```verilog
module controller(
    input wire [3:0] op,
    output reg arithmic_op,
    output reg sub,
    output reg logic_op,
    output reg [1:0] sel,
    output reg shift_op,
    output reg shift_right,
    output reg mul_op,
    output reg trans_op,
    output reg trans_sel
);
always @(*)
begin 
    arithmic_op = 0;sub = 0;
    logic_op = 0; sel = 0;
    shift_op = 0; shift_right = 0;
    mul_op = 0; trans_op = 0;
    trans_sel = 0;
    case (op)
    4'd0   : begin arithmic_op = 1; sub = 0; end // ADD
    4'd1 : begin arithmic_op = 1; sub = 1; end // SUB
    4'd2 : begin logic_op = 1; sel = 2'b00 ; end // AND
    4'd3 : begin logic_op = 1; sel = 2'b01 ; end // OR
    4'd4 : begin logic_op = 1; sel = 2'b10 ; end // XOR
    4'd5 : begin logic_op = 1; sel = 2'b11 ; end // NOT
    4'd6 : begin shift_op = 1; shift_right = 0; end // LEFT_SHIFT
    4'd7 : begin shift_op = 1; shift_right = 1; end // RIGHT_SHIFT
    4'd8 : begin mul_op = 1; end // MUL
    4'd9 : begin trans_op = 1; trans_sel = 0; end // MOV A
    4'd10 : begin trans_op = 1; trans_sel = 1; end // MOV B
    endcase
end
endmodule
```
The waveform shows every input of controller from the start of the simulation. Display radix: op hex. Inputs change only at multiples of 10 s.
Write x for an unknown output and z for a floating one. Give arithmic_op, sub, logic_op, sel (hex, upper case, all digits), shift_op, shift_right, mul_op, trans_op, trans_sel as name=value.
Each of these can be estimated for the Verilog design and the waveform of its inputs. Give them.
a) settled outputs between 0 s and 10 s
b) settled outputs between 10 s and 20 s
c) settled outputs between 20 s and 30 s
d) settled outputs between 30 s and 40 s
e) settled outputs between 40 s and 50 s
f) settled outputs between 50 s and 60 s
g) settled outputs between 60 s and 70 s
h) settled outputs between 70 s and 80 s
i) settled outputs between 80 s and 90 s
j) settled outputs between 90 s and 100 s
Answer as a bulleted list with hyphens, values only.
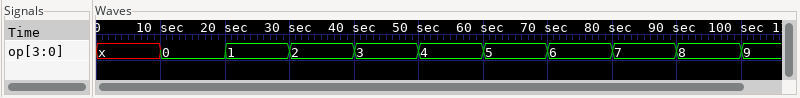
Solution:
- arithmic_op=x, sub=x, logic_op=x, sel=x, shift_op=x, shift_right=x, mul_op=x, trans_op=x, trans_sel=x
- arithmic_op=1, sub=0, logic_op=0, sel=0, shift_op=0, shift_right=0, mul_op=0, trans_op=0, trans_sel=0
- arithmic_op=1, sub=1, logic_op=0, sel=0, shift_op=0, shift_right=0, mul_op=0, trans_op=0, trans_sel=0
- arithmic_op=0, sub=0, logic_op=1, sel=0, shift_op=0, shift_right=0, mul_op=0, trans_op=0, trans_sel=0
- arithmic_op=0, sub=0, logic_op=1, sel=1, shift_op=0, shift_right=0, mul_op=0, trans_op=0, trans_sel=0
- arithmic_op=0, sub=0, logic_op=1, sel=2, shift_op=0, shift_right=0, mul_op=0, trans_op=0, trans_sel=0
- arithmic_op=0, sub=0, logic_op=1, sel=3, shift_op=0, shift_right=0, mul_op=0, trans_op=0, trans_sel=0
- arithmic_op=0, sub=0, logic_op=0, sel=0, shift_op=1, shift_right=0, mul_op=0, trans_op=0, trans_sel=0
- arithmic_op=0, sub=0, logic_op=0, sel=0, shift_op=1, shift_right=1, mul_op=0, trans_op=0, trans_sel=0
- arithmic_op=0, sub=0, logic_op=0, sel=0, shift_op=0, shift_right=0, mul_op=1, trans_op=0, trans_sel=0
